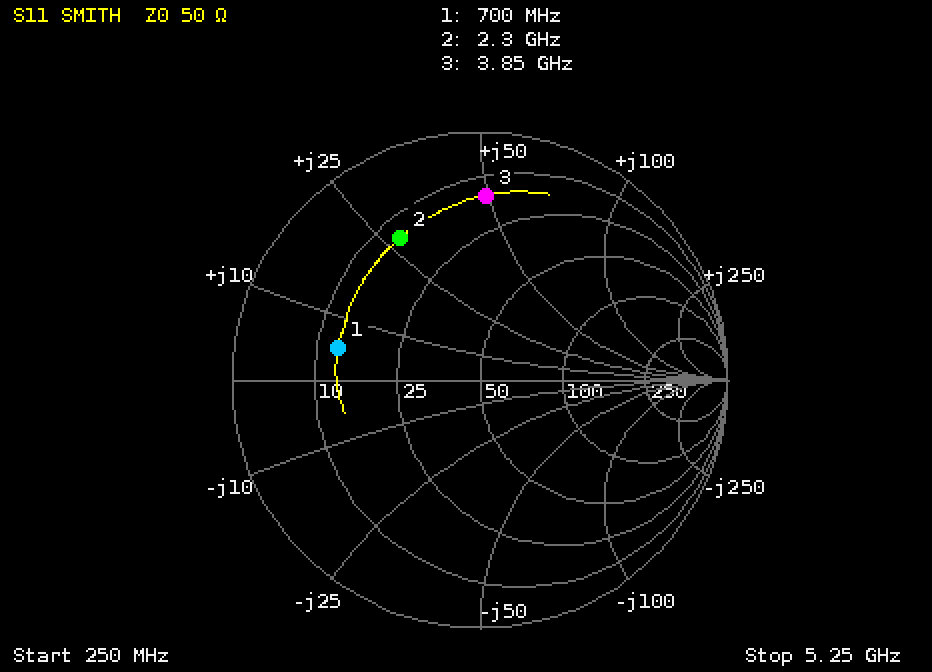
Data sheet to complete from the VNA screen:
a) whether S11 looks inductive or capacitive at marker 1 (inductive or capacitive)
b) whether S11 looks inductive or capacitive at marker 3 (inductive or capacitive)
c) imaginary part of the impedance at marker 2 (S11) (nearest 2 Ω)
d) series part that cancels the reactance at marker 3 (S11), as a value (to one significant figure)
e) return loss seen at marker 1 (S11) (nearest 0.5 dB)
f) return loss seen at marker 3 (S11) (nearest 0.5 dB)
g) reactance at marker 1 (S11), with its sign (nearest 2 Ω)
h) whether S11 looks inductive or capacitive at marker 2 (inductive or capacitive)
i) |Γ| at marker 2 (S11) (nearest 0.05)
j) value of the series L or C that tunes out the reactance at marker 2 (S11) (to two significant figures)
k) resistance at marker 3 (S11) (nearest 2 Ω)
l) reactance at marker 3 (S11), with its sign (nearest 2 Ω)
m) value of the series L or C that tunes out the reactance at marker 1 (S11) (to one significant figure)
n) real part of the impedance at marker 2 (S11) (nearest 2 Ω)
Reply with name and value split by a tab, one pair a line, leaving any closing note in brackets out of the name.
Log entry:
whether S11 looks inductive or capacitive at marker 1	inductive
whether S11 looks inductive or capacitive at marker 3	inductive
imaginary part of the impedance at marker 2 (S11)	+28 Ω
series part that cancels the reactance at marker 3 (S11), as a value	800 fF
return loss seen at marker 1 (S11)	4.5 dB
return loss seen at marker 3 (S11)	2.5 dB
reactance at marker 1 (S11), with its sign	+6 Ω
whether S11 looks inductive or capacitive at marker 2	inductive
|Γ| at marker 2 (S11)	0.65
value of the series L or C that tunes out the reactance at marker 2 (S11)	2.5 pF
resistance at marker 3 (S11)	14 Ω
reactance at marker 3 (S11), with its sign	+50 Ω
value of the series L or C that tunes out the reactance at marker 1 (S11)	40 pF
real part of the impedance at marker 2 (S11)	14 Ω
